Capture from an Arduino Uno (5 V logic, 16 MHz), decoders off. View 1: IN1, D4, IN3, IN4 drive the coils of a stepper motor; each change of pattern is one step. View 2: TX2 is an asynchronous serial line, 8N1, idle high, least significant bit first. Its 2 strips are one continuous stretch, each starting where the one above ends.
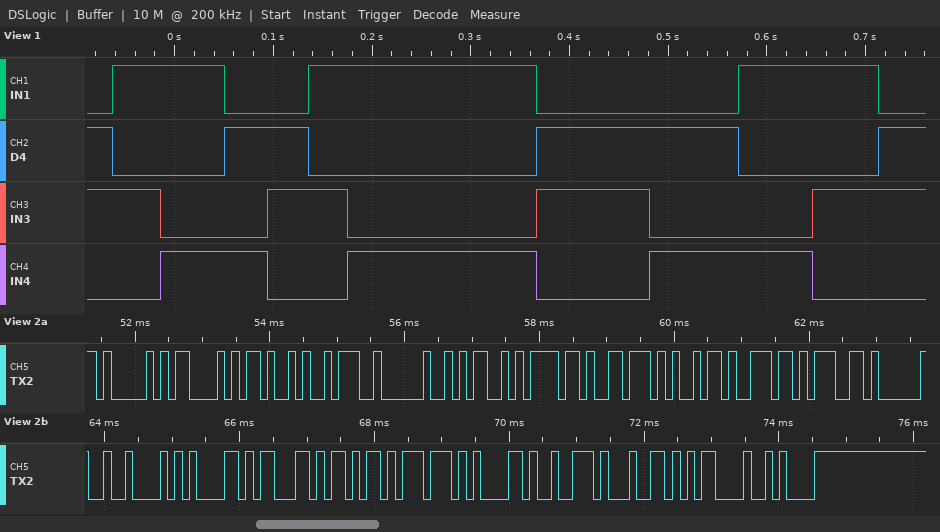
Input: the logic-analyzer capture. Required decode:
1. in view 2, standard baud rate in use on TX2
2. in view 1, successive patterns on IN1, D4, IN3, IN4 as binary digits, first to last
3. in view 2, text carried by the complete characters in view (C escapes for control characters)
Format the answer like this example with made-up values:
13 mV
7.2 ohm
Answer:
9600 baud
0110 1010 1001 0101 0110 1010 1001 0110 0101 1001 1010 0110
"ACK: Moving Backward\r\n"
